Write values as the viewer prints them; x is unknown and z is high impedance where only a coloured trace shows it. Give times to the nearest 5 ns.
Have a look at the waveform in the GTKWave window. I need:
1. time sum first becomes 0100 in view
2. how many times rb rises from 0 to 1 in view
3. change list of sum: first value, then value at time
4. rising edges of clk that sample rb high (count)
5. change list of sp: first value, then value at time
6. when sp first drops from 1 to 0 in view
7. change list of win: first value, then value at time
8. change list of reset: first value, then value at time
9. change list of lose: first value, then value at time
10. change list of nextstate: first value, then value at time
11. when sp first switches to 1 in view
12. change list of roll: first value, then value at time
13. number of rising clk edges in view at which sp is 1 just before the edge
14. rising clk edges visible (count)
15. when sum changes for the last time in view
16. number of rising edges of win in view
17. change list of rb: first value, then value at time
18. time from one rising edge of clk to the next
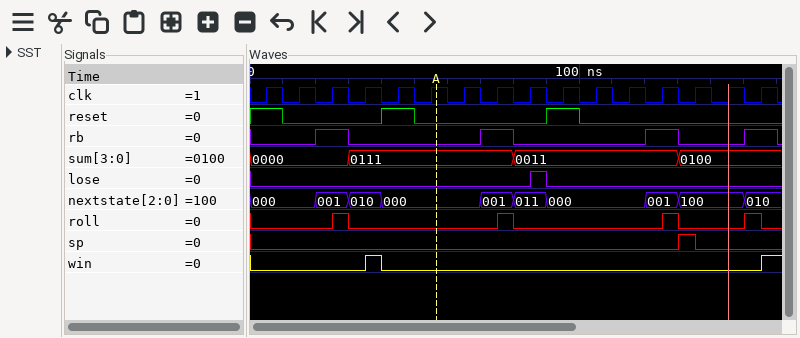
130 ns
4
0000, 0111 at 30 ns, 0011 at 80 ns, 0100 at 130 ns
4
0, 1 at 130 ns, 0 at 135 ns
135 ns
0, 1 at 35 ns, 0 at 40 ns, 1 at 155 ns
1, 0 at 10 ns, 1 at 40 ns, 0 at 50 ns, 1 at 90 ns, 0 at 100 ns
0, 1 at 85 ns, 0 at 90 ns
000, 001 at 20 ns, 010 at 30 ns, 000 at 40 ns, 001 at 70 ns, 011 at 80 ns, 000 at 90 ns, 001 at 120 ns, 100 at 130 ns, 010 at 150 ns
130 ns
0, 1 at 25 ns, 0 at 30 ns, 1 at 75 ns, 0 at 80 ns, 1 at 125 ns, 0 at 130 ns, 1 at 150 ns, 0 at 155 ns
1
16
130 ns
2
0, 1 at 20 ns, 0 at 30 ns, 1 at 70 ns, 0 at 80 ns, 1 at 120 ns, 0 at 130 ns, 1 at 150 ns, 0 at 160 ns
10 ns
